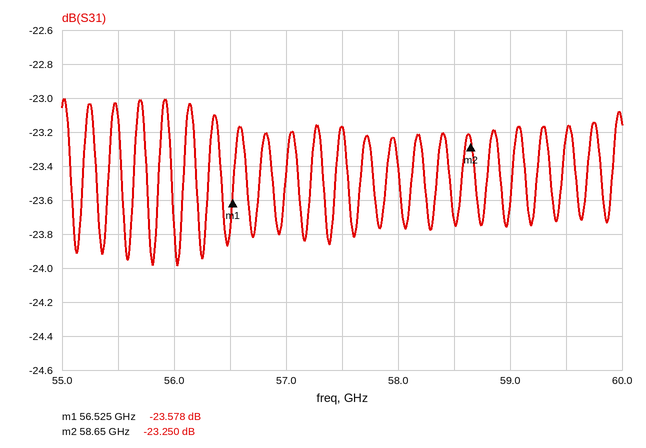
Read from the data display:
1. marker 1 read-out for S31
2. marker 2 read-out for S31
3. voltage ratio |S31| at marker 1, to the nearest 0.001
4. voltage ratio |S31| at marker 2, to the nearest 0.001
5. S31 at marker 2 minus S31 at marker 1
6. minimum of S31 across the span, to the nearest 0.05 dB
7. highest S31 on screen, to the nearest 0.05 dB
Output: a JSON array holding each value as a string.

["-23.578 dB", "-23.250 dB", "0.066", "0.069", "0.328 dB", "-24.00 dB", "-23.00 dB"]
